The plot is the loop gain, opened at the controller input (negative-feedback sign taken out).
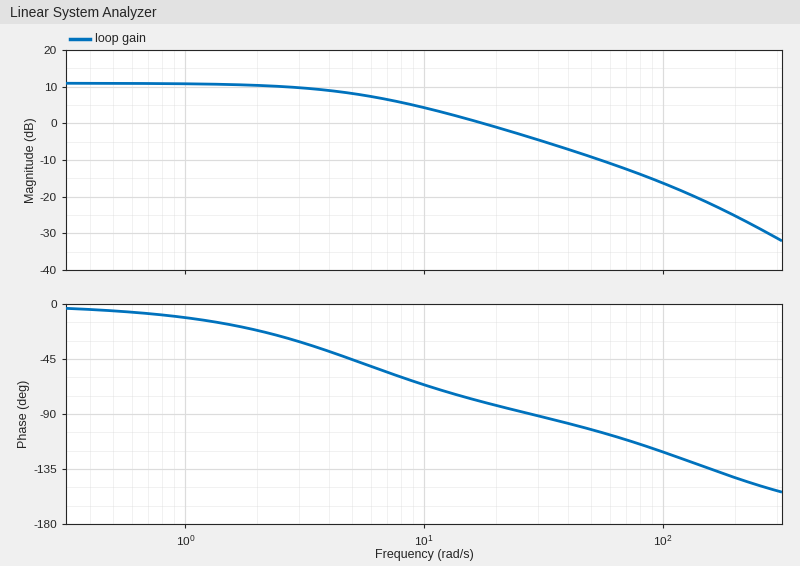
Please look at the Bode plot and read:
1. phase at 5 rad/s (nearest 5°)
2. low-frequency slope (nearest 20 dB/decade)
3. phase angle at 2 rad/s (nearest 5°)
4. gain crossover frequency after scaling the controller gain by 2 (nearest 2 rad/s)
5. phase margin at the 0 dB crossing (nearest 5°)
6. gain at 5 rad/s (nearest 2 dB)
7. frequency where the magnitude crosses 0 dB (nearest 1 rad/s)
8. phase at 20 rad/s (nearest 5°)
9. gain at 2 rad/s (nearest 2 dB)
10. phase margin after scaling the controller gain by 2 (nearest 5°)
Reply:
-45°
0 dB/decade
-20°
36 rad/s
100°
8 dB
18 rad/s
-85°
10 dB
85°
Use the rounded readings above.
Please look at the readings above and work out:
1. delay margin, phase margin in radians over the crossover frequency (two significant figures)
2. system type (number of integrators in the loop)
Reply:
0.097 s
0
